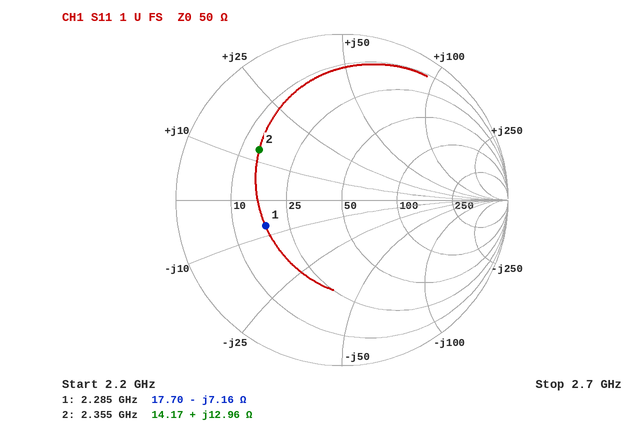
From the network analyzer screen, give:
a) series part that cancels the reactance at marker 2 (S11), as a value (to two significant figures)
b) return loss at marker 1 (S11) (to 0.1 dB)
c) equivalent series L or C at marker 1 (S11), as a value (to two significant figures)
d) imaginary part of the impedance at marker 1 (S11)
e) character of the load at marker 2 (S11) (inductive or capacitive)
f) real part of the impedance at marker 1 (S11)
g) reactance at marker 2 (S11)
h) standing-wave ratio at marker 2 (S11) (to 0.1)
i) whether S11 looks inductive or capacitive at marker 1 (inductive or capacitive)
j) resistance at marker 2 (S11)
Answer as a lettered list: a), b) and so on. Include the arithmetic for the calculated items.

a) C = 1/(2π × 2.355 GHz × 12.96 Ω) ≈ 5.2 pF
b) 6.3 dB
c) C = 1/(2π × 2.285 GHz × 7.16 Ω) ≈ 9.7 pF
d) -7.16 Ω
e) inductive
f) 17.70 Ω
g) +12.96 Ω
h) 3.8
i) capacitive
j) 14.17 Ω
